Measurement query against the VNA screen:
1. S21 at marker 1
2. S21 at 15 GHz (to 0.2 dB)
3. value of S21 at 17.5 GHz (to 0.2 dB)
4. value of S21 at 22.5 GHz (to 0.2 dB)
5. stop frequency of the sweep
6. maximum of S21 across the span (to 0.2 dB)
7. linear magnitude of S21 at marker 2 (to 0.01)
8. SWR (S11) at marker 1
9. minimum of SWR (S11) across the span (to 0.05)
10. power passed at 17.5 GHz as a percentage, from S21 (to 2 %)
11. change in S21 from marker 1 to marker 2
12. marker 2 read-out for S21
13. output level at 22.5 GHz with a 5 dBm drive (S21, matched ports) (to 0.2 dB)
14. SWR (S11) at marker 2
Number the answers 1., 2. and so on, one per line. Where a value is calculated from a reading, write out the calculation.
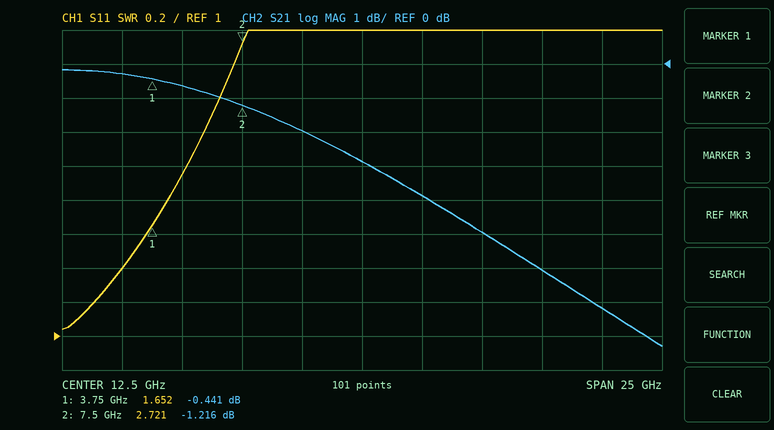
1. -0.441 dB
2. -3.8 dB
3. -5.0 dB
4. -7.2 dB
5. 25 GHz
6. -0.2 dB
7. 10^(-1.216/20) ≈ 0.87
8. 1.652
9. 1.05
10. 10^(-5/10) ≈ 32 %
11. -1.216 − (-0.441) = -0.775 dB
12. -1.216 dB
13. 5 dBm + (-7.2 dB) = -2.2 dBm
14. 2.721
